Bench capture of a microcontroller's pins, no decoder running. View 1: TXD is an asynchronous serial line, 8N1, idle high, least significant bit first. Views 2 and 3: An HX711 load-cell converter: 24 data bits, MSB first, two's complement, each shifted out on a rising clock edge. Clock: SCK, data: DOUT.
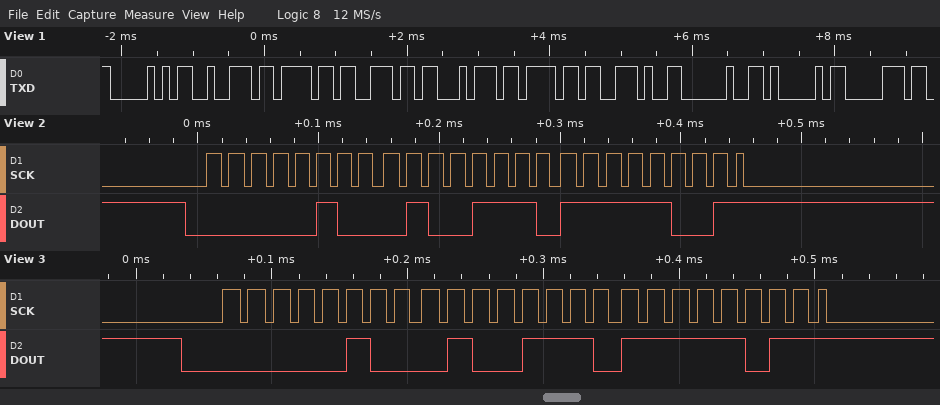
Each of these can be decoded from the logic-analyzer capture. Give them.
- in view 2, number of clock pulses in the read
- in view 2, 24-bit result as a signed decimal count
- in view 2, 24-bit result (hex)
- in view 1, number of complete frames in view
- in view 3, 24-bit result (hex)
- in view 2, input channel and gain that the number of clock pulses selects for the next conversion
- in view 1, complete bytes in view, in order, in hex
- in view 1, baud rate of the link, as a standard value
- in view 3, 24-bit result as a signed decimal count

25
282361
0x044EF9
10
0x044EFB
channel A, gain 128
50 72 6F 6E 74 6F 2E 20 41 70
9600 baud
282363
